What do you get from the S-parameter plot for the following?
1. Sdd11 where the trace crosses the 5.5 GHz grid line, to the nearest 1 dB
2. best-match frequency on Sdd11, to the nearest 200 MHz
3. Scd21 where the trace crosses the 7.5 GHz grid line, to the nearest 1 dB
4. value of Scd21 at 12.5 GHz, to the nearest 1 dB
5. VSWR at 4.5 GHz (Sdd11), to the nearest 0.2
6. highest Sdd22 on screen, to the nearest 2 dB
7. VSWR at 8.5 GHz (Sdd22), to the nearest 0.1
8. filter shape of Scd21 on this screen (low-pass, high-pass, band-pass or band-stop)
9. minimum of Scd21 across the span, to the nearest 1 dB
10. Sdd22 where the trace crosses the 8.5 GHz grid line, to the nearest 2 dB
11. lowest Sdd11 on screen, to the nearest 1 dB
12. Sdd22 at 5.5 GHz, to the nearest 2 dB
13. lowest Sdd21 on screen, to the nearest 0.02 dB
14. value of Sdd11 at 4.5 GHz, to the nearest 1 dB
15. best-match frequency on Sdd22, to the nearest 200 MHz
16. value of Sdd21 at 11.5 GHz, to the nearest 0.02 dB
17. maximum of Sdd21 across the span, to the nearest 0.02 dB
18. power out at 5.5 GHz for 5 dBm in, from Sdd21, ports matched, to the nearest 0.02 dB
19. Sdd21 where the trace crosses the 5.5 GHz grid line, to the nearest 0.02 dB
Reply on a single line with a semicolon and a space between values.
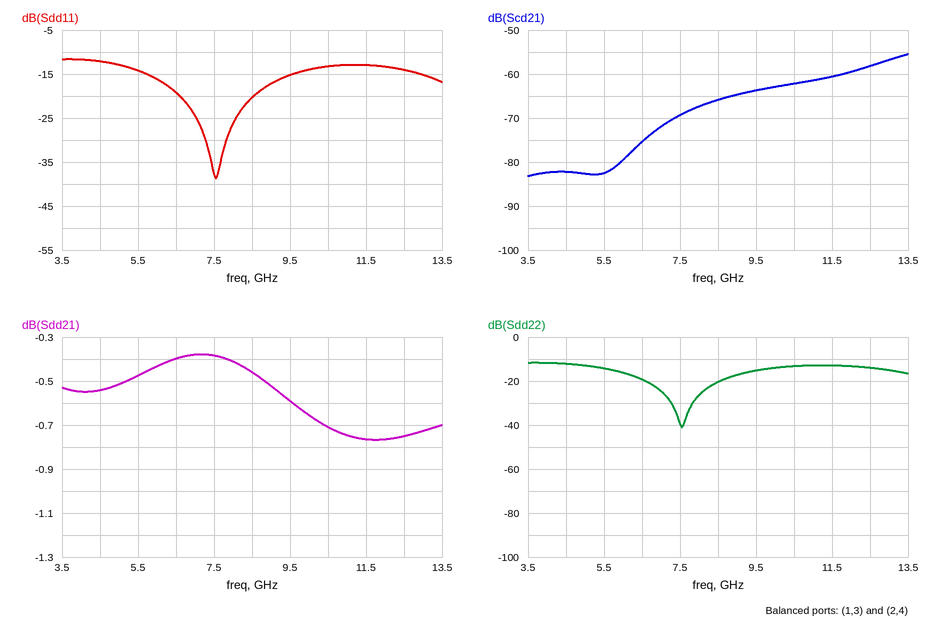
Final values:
-14 dB; 7.6 GHz; -69 dB; -58 dB; 1.6; -12 dB; 1.2; high-pass; -83 dB; -20 dB; -39 dB; -14 dB; -0.76 dB; -12 dB; 7.6 GHz; -0.76 dB; -0.38 dB; 4.52 dBm; -0.48 dB
